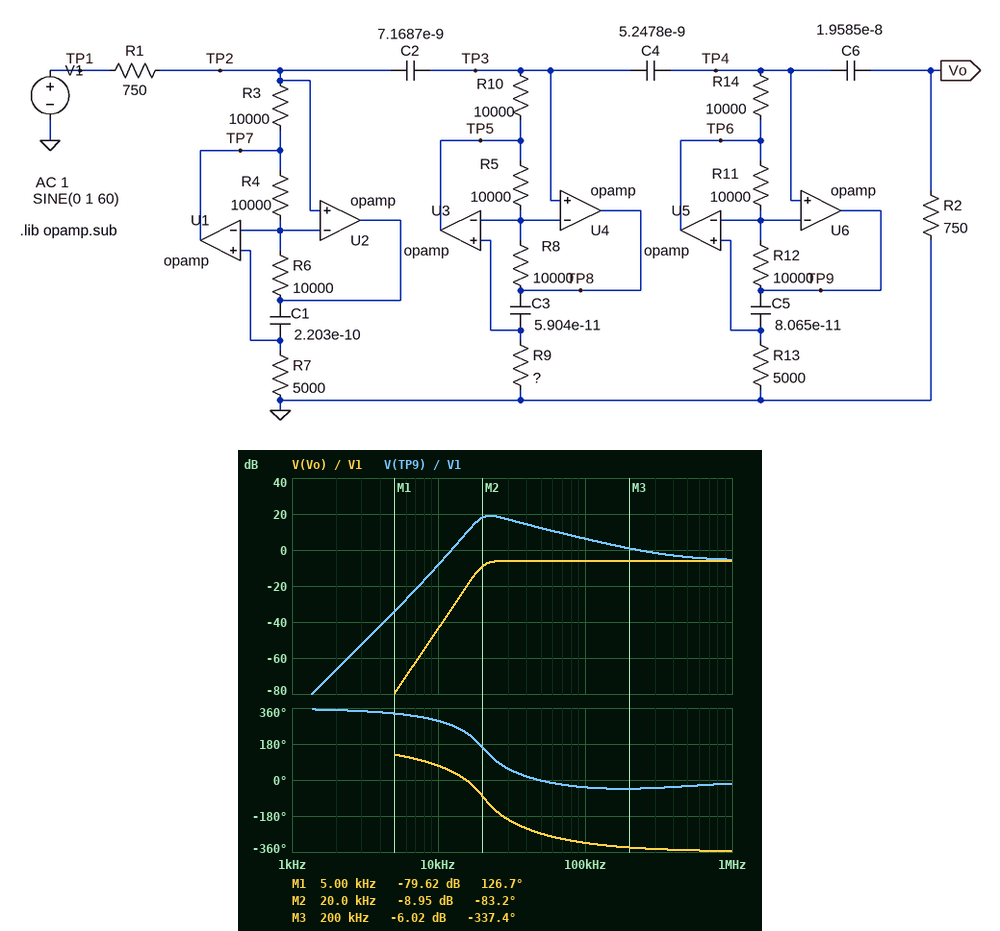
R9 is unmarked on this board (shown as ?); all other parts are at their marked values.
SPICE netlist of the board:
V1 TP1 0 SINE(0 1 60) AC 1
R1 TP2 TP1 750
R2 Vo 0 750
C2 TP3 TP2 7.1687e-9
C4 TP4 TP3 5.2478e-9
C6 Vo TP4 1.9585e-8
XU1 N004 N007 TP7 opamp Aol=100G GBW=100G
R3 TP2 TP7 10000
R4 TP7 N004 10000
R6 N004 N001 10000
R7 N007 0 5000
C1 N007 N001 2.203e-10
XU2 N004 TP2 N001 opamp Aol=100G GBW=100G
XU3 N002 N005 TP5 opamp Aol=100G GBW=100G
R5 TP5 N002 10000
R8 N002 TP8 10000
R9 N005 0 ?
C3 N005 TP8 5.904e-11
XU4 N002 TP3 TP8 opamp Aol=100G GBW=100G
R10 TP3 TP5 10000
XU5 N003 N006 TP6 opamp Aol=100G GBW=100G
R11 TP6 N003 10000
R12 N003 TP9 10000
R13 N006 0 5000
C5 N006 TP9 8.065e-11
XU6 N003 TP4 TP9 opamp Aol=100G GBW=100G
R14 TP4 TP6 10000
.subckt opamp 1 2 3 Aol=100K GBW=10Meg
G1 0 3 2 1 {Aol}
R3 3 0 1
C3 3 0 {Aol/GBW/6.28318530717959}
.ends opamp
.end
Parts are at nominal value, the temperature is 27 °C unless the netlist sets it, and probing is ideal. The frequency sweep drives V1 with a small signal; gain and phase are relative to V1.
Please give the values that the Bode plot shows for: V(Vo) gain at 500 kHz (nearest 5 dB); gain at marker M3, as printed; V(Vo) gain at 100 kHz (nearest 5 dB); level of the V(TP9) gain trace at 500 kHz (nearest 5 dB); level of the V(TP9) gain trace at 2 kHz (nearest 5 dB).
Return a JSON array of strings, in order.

["-5 dB", "-6.02 dB", "-5 dB", "-5 dB", "-65 dB"]
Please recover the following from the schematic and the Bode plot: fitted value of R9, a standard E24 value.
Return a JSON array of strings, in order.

["5.6 kΩ"]
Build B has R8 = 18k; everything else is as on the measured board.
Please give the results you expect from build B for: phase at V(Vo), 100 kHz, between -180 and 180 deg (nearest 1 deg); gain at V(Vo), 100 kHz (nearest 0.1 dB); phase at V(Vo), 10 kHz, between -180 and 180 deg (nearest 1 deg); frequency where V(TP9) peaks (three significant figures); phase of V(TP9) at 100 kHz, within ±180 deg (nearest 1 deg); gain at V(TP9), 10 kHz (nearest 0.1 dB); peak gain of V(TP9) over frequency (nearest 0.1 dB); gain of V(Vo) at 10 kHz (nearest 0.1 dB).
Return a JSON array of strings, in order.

["41 deg", "-6.1 dB", "69 deg", "17.0 kHz", "-41 deg", "-1.2 dB", "21.3 dB", "-36.5 dB"]
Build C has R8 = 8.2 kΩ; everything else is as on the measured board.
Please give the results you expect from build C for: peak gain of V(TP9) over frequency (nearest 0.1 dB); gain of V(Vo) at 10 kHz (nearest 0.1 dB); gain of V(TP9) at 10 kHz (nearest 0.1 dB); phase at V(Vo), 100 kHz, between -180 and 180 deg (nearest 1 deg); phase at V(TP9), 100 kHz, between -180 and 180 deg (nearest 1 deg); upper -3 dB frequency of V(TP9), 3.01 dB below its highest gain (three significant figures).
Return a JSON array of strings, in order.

["17.9 dB", "-45.4 dB", "-10.1 dB", "48 deg", "-34 deg", "37.2 kHz"]
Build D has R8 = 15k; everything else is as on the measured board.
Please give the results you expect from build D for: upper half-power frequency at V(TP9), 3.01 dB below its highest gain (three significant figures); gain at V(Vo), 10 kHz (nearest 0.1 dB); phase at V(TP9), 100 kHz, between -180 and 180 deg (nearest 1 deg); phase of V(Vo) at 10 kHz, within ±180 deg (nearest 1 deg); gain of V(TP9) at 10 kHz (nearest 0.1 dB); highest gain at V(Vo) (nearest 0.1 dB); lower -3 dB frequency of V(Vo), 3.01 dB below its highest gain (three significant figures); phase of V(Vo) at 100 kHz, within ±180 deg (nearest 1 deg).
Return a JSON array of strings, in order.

["26.0 kHz", "-38.8 dB", "-40 deg", "70 deg", "-3.5 dB", "-6.0 dB", "17.0 kHz", "42 deg"]
